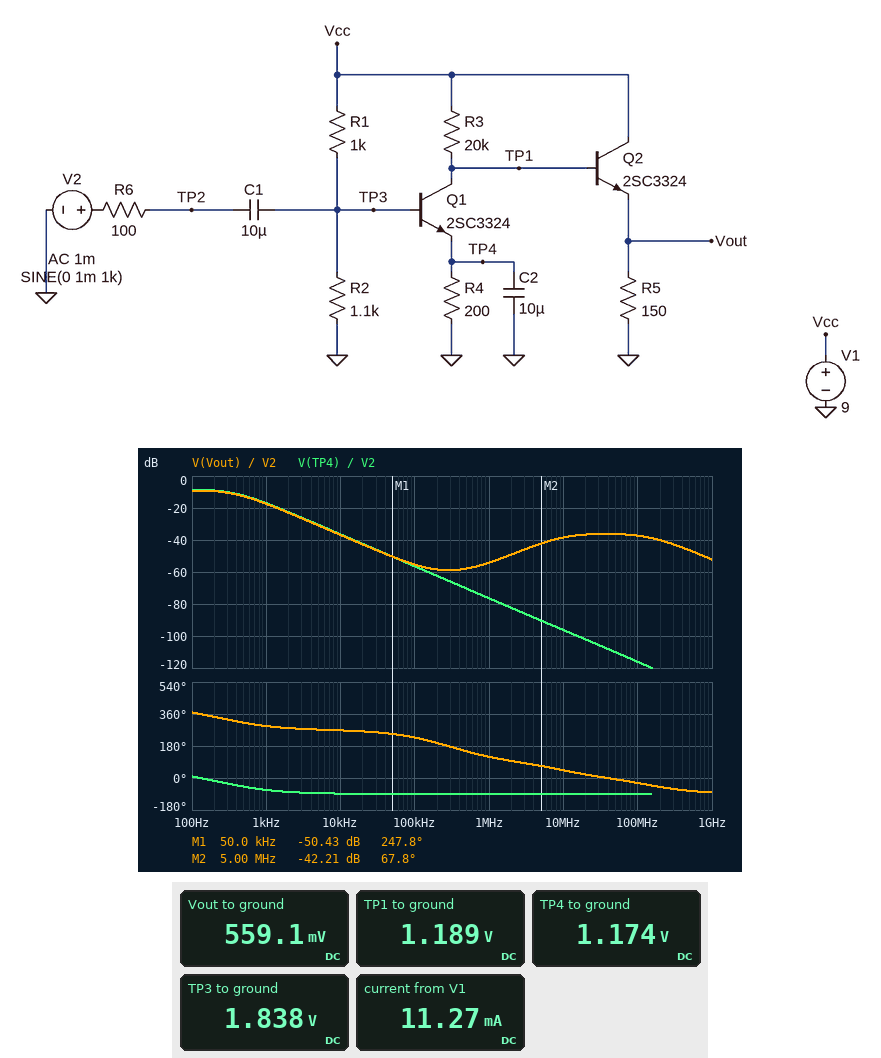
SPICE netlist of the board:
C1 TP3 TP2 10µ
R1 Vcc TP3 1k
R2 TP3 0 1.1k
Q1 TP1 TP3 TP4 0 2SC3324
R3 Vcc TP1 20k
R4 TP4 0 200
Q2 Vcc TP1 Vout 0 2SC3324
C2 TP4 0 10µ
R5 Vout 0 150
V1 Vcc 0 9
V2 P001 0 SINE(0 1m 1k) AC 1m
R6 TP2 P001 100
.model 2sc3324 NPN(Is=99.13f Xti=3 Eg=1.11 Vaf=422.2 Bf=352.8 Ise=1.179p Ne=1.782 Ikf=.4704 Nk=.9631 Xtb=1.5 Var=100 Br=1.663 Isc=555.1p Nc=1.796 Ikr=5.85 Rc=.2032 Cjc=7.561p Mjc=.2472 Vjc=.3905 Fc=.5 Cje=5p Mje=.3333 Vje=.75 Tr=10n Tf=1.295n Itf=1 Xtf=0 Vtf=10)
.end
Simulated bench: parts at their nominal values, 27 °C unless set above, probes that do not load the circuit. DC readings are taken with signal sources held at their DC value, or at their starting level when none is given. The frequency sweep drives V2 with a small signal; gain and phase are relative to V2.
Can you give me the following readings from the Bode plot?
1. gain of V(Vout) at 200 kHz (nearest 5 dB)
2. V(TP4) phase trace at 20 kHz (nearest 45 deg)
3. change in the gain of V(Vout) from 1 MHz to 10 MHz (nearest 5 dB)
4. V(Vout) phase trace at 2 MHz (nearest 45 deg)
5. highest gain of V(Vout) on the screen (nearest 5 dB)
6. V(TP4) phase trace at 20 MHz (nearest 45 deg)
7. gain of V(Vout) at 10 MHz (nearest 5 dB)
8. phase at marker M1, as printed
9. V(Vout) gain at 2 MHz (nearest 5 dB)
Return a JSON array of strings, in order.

["-60 dB", "-90 deg", "15 dB", "90 deg", "-10 dB", "-90 deg", "-40 dB", "247.8 deg", "-50 dB"]
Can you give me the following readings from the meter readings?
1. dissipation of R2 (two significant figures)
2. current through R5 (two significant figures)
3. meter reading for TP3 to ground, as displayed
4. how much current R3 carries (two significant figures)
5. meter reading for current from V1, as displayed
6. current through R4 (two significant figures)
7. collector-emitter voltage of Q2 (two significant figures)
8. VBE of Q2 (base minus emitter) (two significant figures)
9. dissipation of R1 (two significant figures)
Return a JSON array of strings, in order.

["3.1 mW", "3.7 mA", "1.838 V", "390 µA", "11.27 mA", "5.9 mA", "8.4 V", "630 mV", "51 mW"]
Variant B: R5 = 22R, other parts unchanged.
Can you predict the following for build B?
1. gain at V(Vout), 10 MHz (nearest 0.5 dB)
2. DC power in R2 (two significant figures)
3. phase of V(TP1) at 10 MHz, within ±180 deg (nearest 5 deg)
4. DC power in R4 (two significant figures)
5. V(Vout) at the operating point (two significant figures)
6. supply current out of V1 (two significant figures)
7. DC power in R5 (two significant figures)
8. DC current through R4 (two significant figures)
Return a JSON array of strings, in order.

["-38.5 dB", "3.0 mW", "40 deg", "6.8 mW", "500 mV", "30 mA", "11 mW", "5.8 mA"]
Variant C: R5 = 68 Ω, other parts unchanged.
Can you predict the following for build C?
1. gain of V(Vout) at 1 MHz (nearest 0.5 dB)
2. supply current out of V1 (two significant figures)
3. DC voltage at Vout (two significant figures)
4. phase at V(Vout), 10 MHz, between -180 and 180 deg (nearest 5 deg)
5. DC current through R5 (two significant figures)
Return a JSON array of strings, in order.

["-54.5 dB", "15 mA", "540 mV", "45 deg", "7.9 mA"]
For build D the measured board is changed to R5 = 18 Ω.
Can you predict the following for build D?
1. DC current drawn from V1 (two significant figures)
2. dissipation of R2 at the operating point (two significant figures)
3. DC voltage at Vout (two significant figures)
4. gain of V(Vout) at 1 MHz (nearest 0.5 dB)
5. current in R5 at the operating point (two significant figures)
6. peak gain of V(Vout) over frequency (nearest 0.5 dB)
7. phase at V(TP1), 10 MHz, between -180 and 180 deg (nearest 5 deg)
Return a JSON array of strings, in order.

["35 mA", "3.0 mW", "490 mV", "-55.0 dB", "27 mA", "-9.5 dB", "40 deg"]
